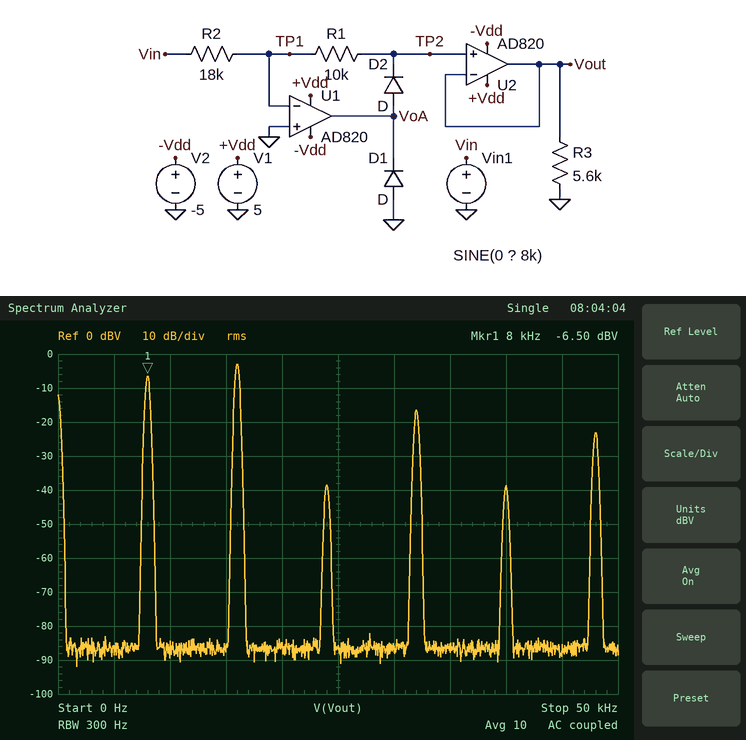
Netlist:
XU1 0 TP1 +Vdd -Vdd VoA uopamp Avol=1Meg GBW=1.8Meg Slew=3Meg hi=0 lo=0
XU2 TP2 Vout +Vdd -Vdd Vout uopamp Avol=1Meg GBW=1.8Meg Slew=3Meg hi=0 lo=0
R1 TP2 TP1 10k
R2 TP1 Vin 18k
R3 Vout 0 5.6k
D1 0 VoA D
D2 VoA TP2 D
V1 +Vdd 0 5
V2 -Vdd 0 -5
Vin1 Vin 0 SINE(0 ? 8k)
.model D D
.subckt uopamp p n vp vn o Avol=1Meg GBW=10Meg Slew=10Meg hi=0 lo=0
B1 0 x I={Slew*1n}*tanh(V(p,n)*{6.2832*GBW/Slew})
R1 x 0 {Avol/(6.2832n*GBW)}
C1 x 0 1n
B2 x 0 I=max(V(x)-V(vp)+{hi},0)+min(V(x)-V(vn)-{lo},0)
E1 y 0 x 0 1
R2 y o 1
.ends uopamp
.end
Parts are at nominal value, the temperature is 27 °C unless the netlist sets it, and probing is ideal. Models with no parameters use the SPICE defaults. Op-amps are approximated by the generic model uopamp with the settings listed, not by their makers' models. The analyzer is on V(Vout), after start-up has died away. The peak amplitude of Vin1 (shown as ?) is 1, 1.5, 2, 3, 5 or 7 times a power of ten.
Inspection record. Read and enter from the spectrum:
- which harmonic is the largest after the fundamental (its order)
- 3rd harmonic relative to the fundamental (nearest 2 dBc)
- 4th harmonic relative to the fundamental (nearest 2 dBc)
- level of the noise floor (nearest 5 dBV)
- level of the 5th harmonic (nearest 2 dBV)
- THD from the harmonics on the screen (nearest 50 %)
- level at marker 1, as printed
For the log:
2
-32 dBc
-10 dBc
-85 dBV
-38 dBV
150 %
-6.50 dBV
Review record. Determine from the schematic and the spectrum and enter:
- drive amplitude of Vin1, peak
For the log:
3 V
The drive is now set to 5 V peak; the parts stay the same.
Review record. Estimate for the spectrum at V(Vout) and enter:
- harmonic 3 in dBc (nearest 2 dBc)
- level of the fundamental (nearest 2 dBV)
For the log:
-34 dBc
-2 dBV
